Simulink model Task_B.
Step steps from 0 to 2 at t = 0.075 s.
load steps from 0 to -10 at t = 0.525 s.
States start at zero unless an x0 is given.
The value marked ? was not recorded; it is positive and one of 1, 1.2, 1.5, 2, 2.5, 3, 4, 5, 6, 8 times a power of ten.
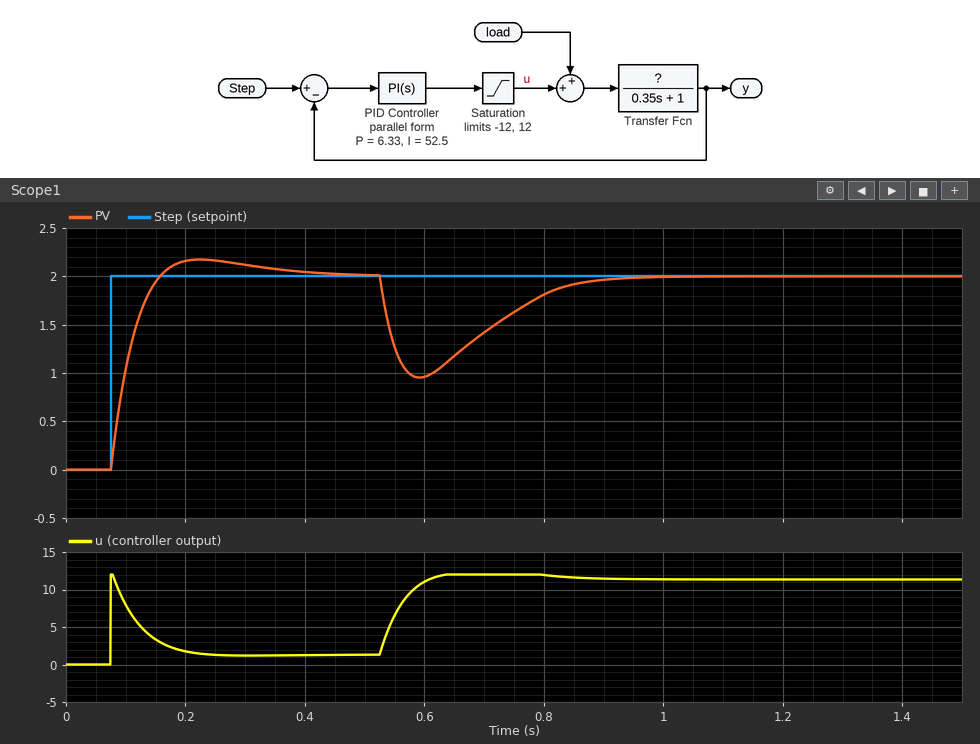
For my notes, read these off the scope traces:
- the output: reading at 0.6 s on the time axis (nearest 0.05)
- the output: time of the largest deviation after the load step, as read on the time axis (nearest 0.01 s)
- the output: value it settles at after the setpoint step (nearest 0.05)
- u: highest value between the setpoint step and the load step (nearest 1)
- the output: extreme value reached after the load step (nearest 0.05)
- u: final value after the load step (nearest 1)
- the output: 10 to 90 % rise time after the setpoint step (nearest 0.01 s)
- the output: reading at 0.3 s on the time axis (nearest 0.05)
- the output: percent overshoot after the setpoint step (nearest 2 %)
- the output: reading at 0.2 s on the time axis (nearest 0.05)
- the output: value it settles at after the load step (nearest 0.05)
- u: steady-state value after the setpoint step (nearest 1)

0.95
0.59 s
2.00
12
0.95
11
0.06 s
2.10
8 %
2.15
2.00
1
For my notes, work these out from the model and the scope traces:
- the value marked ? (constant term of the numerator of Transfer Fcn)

1.5
